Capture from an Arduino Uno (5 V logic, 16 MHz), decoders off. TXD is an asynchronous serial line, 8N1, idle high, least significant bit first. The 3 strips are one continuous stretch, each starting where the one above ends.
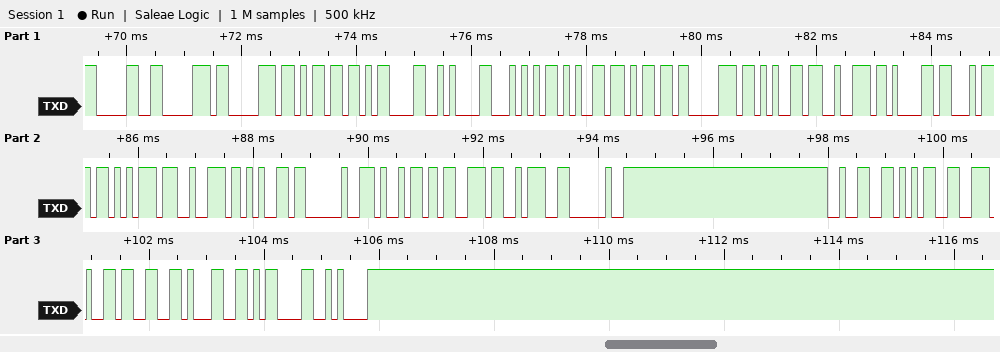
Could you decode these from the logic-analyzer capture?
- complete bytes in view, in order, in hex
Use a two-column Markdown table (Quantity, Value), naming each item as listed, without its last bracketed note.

| Quantity | Value |
|---|---|
| complete bytes in view, in order, in hex | 0x30 0x70 0x70 0x6D 0x0D 0x0A 0x54 0x65 0x6D 0x70 0x65 0x72 0x61 0x74 0x75 0x72 0x65 0x20 0x69 0x73 0x3A 0x20 0x32 0x35 0x2E 0x33 0x31 0x0D 0x0A |
